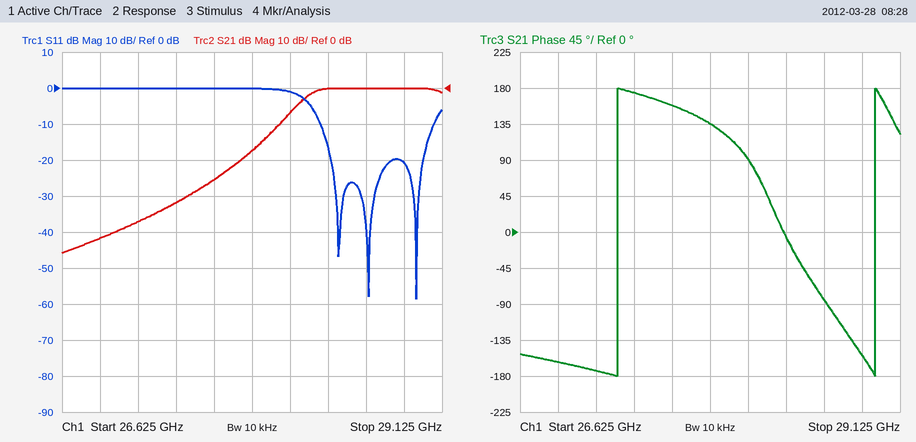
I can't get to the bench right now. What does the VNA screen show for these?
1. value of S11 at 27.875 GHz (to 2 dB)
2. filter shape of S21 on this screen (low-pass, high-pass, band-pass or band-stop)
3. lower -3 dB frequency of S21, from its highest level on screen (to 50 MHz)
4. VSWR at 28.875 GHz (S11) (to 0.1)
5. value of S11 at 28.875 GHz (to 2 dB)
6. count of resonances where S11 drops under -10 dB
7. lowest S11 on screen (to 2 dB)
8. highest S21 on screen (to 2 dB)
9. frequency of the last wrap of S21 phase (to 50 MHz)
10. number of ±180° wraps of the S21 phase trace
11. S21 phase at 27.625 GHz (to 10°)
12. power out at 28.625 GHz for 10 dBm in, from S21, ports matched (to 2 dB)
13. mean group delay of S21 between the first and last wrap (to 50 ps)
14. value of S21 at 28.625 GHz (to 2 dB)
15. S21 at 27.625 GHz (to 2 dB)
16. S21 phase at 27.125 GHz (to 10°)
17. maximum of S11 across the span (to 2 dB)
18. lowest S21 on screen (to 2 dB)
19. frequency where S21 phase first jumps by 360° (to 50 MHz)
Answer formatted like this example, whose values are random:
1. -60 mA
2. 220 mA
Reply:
1. 0 dB
2. high-pass
3. 28.20 GHz
4. 1.2
5. -20 dB
6. 3
7. -58 dB
8. 0 dB
9. 28.95 GHz
10. 2
11. 160°
12. 10 dBm
13. 600 ps
14. 0 dB
15. -26 dB
16. -170°
17. 0 dB
18. -46 dB
19. 27.25 GHz
